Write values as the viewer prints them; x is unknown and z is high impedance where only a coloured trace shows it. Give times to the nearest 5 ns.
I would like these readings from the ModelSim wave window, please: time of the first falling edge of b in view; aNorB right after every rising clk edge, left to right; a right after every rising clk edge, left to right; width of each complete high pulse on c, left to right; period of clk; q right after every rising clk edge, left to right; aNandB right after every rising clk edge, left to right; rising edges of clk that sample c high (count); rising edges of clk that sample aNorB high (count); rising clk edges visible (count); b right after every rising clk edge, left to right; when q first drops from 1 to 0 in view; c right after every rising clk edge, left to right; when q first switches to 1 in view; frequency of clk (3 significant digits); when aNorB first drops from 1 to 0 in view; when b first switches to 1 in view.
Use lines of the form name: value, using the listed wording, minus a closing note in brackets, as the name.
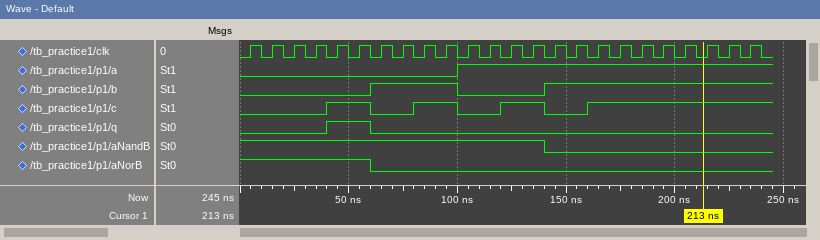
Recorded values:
time of the first falling edge of b in view: 100 ns
aNorB right after every rising clk edge, left to right: 1 1 1 1 1 1 0 0 0 0 0 0 0 0 0 0 0 0 0 0 0 0 0 0
a right after every rising clk edge, left to right: 0 0 0 0 0 0 0 0 0 0 1 1 1 1 1 1 1 1 1 1 1 1 1 1
width of each complete high pulse on c, left to right: 20 ns, 20 ns, 20 ns
period of clk: 10 ns
q right after every rising clk edge, left to right: 0 0 0 0 1 1 0 0 0 0 0 0 0 0 0 0 0 0 0 0 0 0 0 0
aNandB right after every rising clk edge, left to right: 1 1 1 1 1 1 1 1 1 1 1 1 1 1 0 0 0 0 0 0 0 0 0 0
rising edges of clk that sample c high: 14
rising edges of clk that sample aNorB high: 6
rising clk edges visible: 24
b right after every rising clk edge, left to right: 0 0 0 0 0 0 1 1 1 1 0 0 0 0 1 1 1 1 1 1 1 1 1 1
when q first drops from 1 to 0 in view: 60 ns
c right after every rising clk edge, left to right: 0 0 0 0 1 1 0 0 1 1 0 0 1 1 0 0 1 1 1 1 1 1 1 1
when q first switches to 1 in view: 40 ns
frequency of clk: 100 MHz
when aNorB first drops from 1 to 0 in view: 60 ns
when b first switches to 1 in view: 60 ns
